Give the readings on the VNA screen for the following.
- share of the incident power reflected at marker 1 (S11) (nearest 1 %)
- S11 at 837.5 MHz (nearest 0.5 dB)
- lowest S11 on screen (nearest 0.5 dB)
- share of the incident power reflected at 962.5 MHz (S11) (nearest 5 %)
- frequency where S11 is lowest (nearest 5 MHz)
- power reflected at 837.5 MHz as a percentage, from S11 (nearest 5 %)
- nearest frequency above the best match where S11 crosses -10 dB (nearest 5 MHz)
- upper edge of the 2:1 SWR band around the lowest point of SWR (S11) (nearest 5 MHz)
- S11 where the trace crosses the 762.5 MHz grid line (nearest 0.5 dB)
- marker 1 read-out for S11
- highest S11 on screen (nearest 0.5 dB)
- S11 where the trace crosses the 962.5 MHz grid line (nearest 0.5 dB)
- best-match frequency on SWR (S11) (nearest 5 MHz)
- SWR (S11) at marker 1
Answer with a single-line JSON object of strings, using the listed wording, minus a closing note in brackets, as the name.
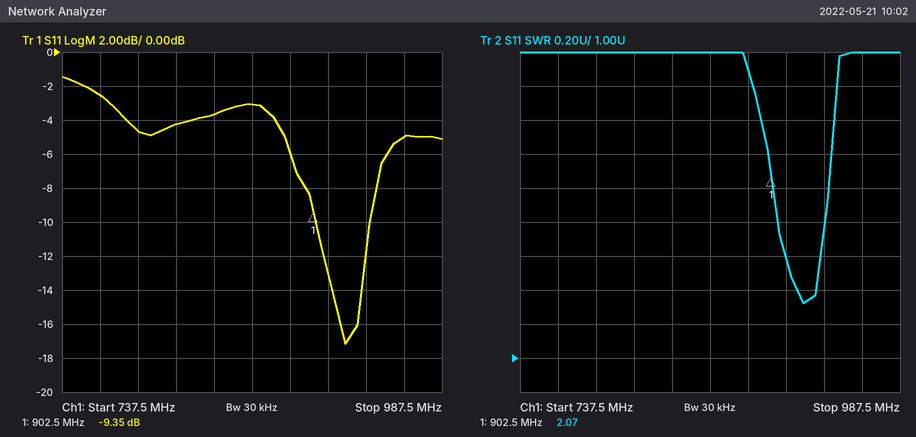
{"share of the incident power reflected at marker 1 (S11)": "12 %", "S11 at 837.5 MHz": "-3.5 dB", "lowest S11 on screen": "-17.0 dB", "share of the incident power reflected at 962.5 MHz (S11)": "30 %", "frequency where S11 is lowest": "925 MHz", "power reflected at 837.5 MHz as a percentage, from S11": "45 %", "nearest frequency above the best match where S11 crosses -10 dB": "940 MHz", "upper edge of the 2:1 SWR band around the lowest point of SWR (S11)": "940 MHz", "S11 where the trace crosses the 762.5 MHz grid line": "-2.5 dB", "marker 1 read-out for S11": "-9.35 dB", "highest S11 on screen": "-1.5 dB", "S11 where the trace crosses the 962.5 MHz grid line": "-5.0 dB", "best-match frequency on SWR (S11)": "925 MHz", "SWR (S11) at marker 1": "2.07"}
